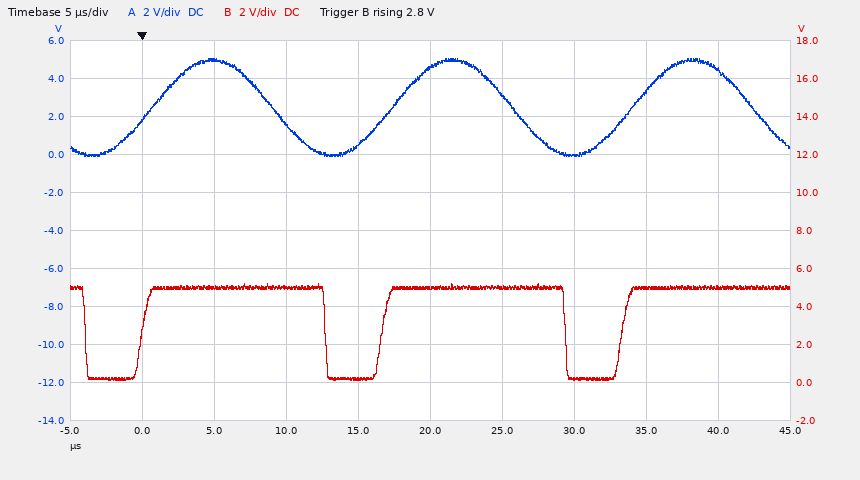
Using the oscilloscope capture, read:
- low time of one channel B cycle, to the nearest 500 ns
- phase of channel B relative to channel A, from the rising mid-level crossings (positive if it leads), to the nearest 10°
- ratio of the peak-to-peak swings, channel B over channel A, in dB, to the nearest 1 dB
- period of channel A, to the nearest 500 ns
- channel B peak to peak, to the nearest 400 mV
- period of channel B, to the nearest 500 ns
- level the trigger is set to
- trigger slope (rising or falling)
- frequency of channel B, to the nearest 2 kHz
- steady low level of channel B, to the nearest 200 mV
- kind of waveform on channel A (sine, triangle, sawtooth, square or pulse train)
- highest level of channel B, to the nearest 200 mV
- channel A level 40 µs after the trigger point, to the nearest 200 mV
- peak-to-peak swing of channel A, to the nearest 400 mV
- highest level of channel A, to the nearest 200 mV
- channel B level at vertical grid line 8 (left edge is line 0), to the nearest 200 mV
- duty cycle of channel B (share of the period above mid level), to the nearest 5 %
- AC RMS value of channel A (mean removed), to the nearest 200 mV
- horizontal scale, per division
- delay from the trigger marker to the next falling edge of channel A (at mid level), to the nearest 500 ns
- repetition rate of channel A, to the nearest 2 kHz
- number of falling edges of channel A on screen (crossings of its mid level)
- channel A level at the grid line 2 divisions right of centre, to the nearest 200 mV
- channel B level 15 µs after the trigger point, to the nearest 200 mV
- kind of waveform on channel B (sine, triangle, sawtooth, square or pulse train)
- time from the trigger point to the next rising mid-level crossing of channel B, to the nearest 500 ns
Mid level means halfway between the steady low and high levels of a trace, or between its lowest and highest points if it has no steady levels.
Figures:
4.0 µs
+20°
0 dB
16.5 µs
5.2 V
16.5 µs
2.8 V
rising
60 kHz
200 mV
sine
5.2 V
4.4 V
5.2 V
5.0 V
5.0 V
75 %
1.8 V
5 µs
9.0 µs
60 kHz
3
0.0 V
200 mV
pulse train
16.5 µs
